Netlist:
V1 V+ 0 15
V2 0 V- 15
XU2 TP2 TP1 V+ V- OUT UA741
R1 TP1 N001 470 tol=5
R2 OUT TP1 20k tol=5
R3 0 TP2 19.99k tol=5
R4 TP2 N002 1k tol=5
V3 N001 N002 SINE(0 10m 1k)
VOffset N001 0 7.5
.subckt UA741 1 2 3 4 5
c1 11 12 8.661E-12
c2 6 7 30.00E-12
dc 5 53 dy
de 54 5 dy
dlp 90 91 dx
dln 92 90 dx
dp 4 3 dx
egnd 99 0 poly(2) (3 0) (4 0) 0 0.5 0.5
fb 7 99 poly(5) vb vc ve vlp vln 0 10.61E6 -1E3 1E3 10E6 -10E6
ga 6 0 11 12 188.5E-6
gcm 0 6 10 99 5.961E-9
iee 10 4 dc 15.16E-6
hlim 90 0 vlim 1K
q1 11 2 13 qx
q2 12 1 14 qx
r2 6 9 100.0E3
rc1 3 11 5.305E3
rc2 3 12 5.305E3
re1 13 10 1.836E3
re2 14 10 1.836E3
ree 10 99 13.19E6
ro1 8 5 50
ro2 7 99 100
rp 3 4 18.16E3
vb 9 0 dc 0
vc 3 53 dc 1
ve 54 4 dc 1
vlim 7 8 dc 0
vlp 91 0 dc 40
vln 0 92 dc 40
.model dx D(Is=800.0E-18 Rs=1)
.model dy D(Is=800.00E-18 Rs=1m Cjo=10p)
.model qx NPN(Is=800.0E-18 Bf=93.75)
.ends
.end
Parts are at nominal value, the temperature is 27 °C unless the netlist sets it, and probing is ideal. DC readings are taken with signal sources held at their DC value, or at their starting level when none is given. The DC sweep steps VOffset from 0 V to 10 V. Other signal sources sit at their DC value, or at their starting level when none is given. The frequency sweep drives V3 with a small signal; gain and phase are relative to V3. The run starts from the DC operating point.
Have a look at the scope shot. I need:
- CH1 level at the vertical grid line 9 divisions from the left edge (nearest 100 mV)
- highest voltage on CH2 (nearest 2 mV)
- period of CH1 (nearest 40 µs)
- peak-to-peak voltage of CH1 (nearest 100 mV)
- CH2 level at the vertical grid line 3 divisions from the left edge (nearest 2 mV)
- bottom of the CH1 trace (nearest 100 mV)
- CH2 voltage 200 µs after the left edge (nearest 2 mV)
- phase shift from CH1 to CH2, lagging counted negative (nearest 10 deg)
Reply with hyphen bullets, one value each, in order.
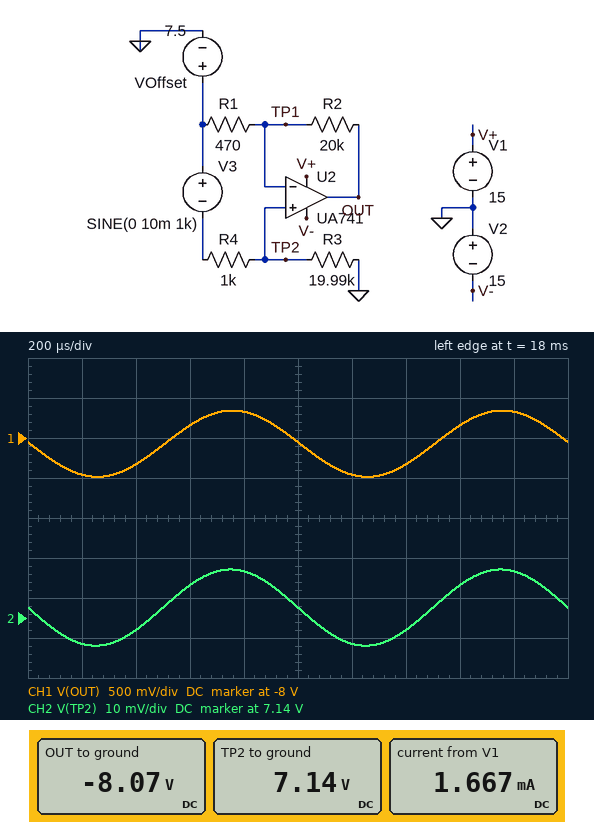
- -7.7 V
- 7.152 V
- 1.00 ms
- 800 mV
- 7.148 V
- -8.5 V
- 7.134 V
- 0 deg
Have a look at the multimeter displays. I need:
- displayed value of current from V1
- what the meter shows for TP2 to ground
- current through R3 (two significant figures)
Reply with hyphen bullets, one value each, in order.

- 1.667 mA
- 7.14 V
- 360 µA
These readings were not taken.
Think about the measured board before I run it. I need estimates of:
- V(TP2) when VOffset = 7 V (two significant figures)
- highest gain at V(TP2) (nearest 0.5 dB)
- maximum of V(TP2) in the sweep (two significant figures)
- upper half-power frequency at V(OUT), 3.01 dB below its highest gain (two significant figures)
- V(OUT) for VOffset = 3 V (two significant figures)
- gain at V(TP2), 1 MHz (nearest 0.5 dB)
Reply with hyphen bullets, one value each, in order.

- 6.7 V
- -0.5 dB
- 9.5 V
- 24 kHz
- -3.2 V
- -0.5 dB
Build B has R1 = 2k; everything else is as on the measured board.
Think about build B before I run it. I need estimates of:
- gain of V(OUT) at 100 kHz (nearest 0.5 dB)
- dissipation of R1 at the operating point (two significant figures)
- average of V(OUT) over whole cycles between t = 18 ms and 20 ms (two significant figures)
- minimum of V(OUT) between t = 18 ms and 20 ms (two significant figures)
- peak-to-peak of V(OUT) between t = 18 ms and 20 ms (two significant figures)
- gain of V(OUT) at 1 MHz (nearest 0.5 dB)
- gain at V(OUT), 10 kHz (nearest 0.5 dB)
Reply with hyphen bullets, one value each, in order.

- 17.5 dB
- 64 µW
- 3.6 V
- 3.5 V
- 210 mV
- -1.0 dB
- 20.5 dB
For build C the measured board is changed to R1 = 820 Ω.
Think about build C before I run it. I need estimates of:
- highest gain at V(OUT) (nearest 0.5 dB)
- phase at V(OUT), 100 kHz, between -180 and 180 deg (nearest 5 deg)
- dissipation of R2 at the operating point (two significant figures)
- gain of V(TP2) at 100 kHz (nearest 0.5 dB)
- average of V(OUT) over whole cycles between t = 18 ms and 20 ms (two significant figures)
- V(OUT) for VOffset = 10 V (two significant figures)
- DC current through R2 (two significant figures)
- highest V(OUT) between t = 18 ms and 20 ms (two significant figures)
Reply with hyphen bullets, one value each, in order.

- 27.5 dB
- 110 deg
- 3.8 mW
- -0.5 dB
- -1.6 V
- -2.1 V
- 440 µA
- -1.3 V
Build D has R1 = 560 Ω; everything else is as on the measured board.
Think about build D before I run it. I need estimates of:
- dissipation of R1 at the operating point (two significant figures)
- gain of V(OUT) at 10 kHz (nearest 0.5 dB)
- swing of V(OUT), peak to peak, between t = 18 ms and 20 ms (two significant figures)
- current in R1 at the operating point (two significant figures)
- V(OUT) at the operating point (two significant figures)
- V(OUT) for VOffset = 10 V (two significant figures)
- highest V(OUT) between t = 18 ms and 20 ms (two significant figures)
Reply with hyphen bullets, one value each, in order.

- 230 µW
- 30.5 dB
- 700 mV
- 640 µA
- -5.6 V
- -7.5 V
- -5.3 V
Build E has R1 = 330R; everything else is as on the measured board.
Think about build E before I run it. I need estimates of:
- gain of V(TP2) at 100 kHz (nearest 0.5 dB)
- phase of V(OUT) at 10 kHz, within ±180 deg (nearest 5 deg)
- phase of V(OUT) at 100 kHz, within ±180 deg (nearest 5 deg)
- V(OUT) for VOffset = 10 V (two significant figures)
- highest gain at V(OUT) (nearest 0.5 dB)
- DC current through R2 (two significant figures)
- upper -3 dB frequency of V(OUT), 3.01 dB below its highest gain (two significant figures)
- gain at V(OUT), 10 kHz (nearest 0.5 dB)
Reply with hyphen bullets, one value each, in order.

- -0.5 dB
- 150 deg
- 95 deg
- -15 V
- 35.5 dB
- 1.1 mA
- 17 kHz
- 34.0 dB
